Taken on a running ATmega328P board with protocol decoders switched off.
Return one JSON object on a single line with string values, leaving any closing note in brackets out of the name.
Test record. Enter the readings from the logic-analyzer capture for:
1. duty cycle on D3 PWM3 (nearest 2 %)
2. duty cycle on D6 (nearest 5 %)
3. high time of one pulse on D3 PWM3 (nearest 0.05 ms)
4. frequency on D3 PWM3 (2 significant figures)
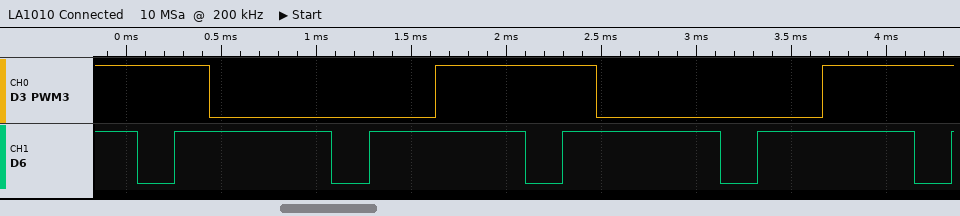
{"duty cycle on D3 PWM3": "42 %", "duty cycle on D6": "80 %", "high time of one pulse on D3 PWM3": "0.85 ms", "frequency on D3 PWM3": "490 Hz"}
